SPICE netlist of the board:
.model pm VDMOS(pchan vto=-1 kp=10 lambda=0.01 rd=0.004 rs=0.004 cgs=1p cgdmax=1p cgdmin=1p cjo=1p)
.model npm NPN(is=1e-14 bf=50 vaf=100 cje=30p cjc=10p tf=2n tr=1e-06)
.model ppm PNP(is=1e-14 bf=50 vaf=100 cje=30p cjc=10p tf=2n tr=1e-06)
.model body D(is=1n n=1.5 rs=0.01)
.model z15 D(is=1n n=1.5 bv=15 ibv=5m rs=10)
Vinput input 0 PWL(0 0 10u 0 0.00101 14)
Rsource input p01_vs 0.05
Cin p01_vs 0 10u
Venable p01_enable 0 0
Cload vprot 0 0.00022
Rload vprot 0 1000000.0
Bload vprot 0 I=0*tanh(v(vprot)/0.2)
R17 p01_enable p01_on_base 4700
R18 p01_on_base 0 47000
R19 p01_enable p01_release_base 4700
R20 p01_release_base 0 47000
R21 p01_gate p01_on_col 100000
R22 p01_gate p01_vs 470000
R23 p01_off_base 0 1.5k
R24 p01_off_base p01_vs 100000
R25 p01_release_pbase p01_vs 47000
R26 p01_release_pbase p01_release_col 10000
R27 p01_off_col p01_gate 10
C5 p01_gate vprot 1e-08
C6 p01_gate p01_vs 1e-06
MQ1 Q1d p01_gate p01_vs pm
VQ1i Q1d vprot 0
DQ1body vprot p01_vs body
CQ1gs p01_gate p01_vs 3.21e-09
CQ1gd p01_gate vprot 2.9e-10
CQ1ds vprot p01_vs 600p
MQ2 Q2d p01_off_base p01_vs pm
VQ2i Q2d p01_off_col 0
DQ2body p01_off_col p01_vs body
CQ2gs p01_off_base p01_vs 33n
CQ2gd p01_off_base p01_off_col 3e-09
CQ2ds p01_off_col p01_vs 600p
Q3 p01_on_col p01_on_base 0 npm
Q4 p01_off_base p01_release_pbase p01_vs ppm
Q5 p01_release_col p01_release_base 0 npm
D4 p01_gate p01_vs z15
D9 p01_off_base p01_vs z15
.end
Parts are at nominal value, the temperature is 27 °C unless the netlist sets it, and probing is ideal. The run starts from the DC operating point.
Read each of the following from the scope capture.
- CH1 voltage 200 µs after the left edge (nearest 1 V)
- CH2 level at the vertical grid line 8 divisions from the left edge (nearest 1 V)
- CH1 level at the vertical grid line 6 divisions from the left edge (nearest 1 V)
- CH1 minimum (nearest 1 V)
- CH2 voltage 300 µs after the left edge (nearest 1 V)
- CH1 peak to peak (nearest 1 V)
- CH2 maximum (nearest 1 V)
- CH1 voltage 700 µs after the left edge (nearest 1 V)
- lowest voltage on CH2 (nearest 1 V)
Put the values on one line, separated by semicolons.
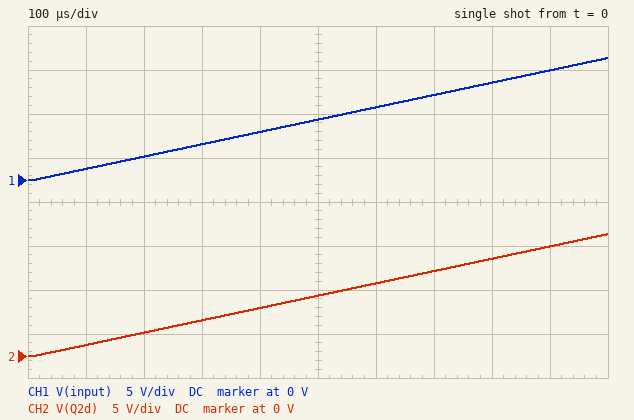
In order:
3 V; 11 V; 8 V; 0 V; 4 V; 14 V; 14 V; 10 V; 0 V
